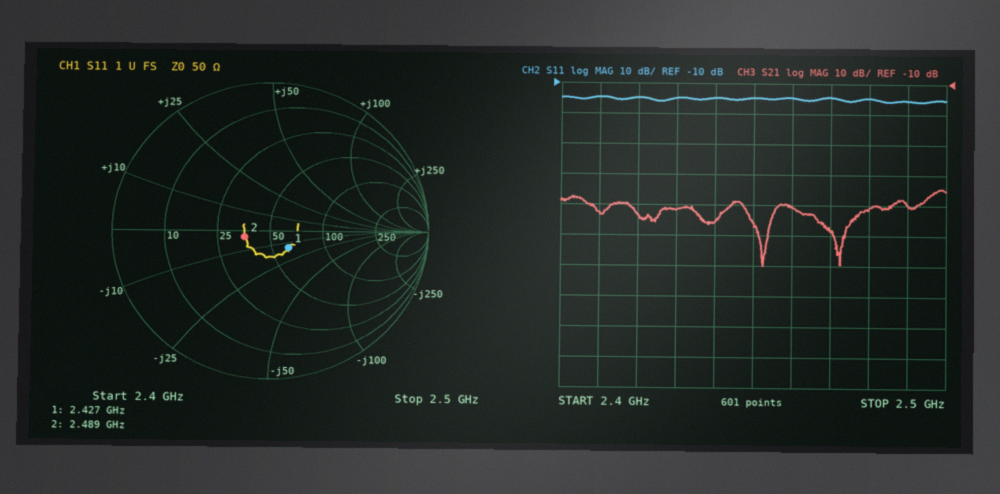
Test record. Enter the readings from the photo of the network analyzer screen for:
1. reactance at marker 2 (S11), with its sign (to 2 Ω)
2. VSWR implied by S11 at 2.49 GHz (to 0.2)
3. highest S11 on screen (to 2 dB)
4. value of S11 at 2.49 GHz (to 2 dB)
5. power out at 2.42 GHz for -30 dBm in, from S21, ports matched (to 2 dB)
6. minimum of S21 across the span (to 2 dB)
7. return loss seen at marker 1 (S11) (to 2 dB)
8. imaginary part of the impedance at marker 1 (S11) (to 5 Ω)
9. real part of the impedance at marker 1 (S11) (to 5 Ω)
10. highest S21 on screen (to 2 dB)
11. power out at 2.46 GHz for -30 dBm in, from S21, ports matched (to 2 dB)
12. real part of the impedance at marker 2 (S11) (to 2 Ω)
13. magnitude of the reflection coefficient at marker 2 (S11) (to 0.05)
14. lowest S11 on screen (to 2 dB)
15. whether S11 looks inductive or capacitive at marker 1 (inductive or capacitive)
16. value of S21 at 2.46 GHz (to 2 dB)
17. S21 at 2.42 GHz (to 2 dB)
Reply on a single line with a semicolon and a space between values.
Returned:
-4 Ω; 1.4; -14 dB; -16 dB; -84 dBm; -70 dB; 16 dB; -15 Ω; 60 Ω; -44 dB; -80 dBm; 36 Ω; 0.15; -16 dB; capacitive; -50 dB; -54 dB
